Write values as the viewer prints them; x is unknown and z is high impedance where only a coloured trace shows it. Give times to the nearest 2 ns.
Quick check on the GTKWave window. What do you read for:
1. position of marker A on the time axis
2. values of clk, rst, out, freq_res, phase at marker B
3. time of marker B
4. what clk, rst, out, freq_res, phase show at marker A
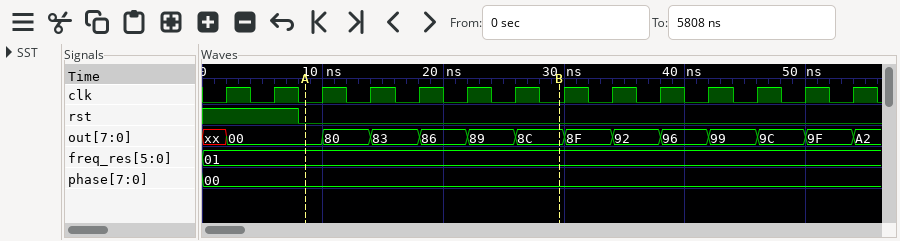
8 ns
clk=0, rst=0, out=8C, freq_res=01, phase=00
30 ns
clk=0, rst=0, out=00, freq_res=01, phase=00
